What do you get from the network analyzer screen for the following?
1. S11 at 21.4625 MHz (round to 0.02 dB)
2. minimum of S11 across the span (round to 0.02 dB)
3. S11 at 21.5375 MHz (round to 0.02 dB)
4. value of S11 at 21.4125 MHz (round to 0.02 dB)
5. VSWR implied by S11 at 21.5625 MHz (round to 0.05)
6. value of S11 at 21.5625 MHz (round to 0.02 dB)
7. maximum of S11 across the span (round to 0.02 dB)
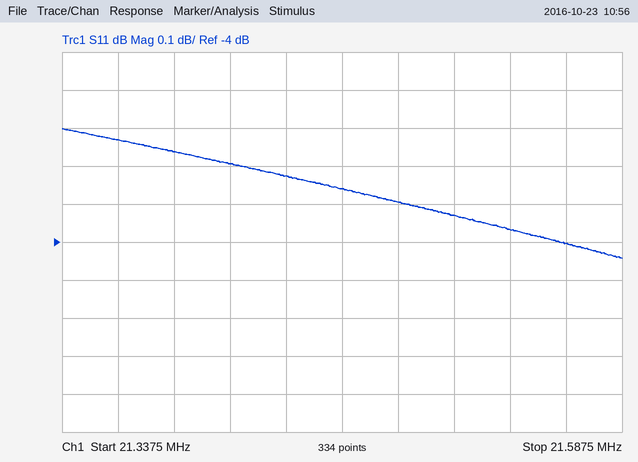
-3.86 dB
-4.04 dB
-3.96 dB
-3.80 dB
4.40
-4.00 dB
-3.70 dB
